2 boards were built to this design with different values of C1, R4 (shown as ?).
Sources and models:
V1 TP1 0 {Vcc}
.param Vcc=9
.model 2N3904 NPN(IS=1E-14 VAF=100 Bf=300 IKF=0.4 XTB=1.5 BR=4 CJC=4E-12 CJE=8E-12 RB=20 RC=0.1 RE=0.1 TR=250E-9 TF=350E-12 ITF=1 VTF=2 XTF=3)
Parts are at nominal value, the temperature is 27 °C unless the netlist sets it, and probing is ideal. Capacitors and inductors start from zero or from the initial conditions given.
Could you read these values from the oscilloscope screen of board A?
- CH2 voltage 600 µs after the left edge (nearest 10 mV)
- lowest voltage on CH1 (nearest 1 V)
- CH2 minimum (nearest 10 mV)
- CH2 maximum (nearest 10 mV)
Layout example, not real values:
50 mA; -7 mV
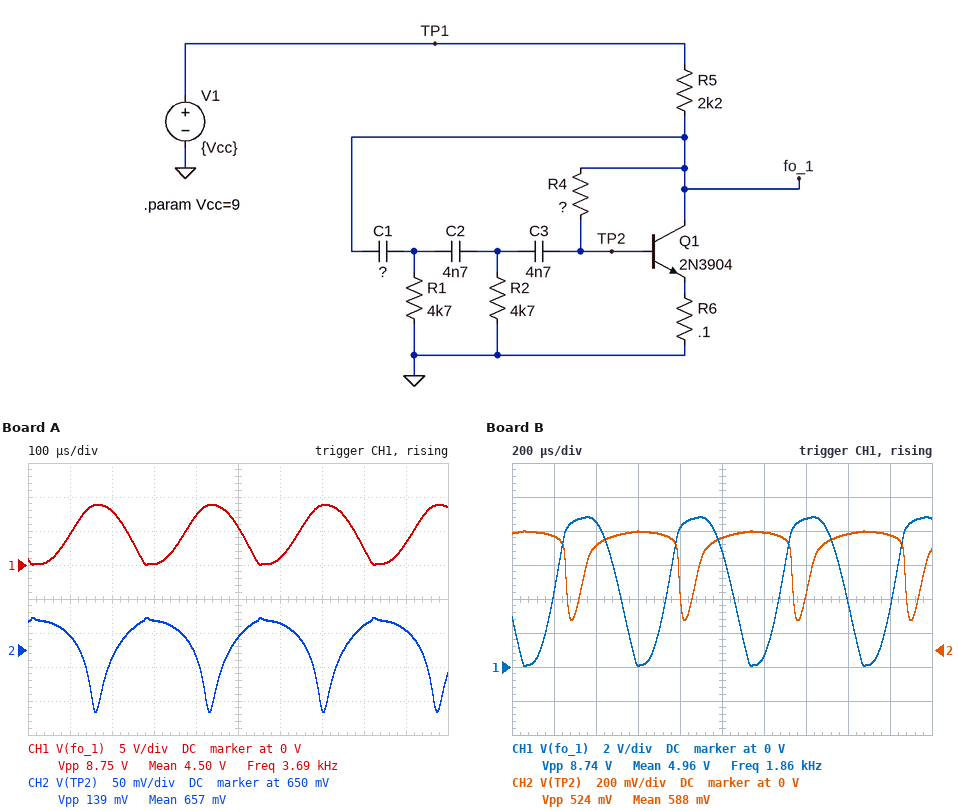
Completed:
690 mV; 0 V; 560 mV; 700 mV
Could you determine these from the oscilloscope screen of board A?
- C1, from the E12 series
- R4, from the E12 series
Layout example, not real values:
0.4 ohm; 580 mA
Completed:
1.8 nF; 390 kΩ
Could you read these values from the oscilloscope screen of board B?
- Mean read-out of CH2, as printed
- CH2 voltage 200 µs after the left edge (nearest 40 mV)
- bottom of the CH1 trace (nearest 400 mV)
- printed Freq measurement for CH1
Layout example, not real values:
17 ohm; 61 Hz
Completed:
588 mV; 680 mV; 0 V; 1.86 kHz
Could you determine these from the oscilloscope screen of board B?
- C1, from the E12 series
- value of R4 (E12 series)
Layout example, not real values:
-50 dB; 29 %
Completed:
8.2 nF; 560 kΩ
